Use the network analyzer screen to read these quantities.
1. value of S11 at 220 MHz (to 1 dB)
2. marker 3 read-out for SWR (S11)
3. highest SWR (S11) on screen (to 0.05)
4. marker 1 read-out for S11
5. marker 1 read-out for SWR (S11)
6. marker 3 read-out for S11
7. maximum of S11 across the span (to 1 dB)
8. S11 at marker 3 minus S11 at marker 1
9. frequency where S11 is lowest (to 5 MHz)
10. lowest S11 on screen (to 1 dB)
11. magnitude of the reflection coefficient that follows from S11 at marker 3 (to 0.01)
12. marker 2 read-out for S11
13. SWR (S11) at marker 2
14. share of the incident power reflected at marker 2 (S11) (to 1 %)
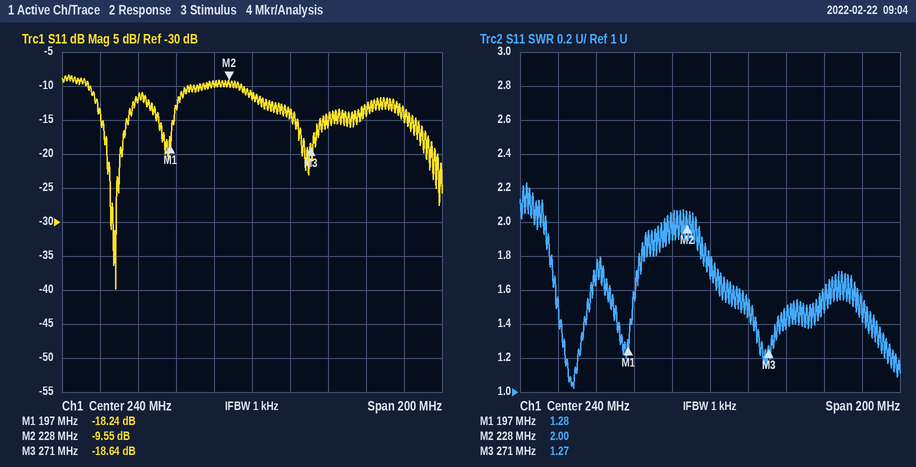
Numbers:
-10 dB
1.27
2.25
-18.24 dB
1.28
-18.64 dB
-8 dB
-0.40 dB
170 MHz
-40 dB
0.12
-9.55 dB
2.00
11 %
